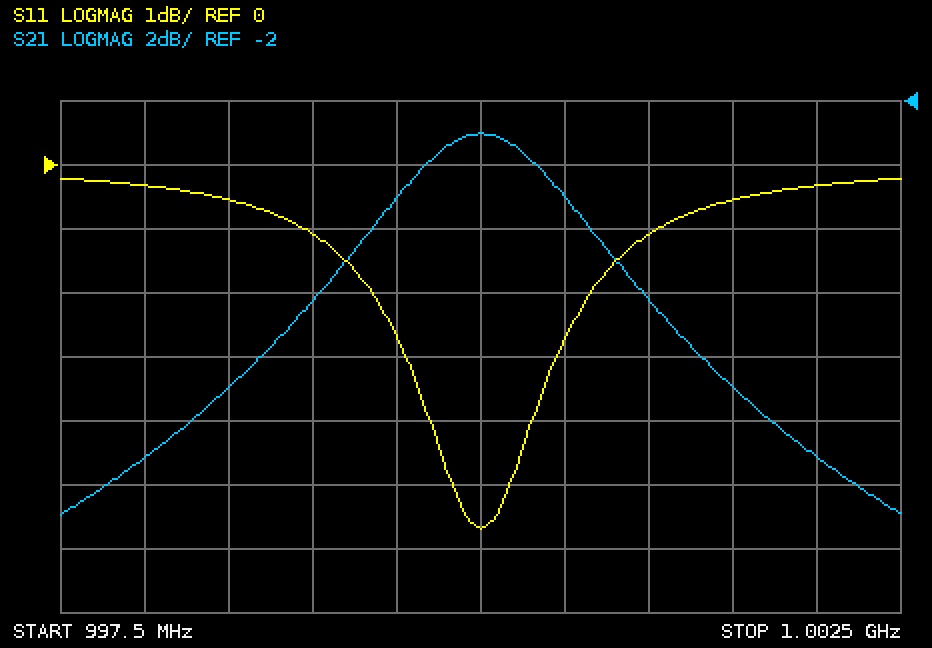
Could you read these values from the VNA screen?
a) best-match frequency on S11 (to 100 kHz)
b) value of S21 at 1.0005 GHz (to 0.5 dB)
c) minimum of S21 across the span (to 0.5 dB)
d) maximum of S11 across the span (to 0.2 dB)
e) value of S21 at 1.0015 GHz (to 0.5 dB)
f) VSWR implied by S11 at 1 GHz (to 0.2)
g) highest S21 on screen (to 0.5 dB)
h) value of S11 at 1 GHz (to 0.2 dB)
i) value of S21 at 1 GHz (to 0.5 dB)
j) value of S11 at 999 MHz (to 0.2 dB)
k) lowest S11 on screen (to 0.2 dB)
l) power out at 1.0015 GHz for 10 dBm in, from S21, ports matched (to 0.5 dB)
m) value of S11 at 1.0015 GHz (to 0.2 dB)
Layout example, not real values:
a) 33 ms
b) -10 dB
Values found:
a) 1.0000 GHz
b) -5.0 dB
c) -15.0 dB
d) -0.2 dB
e) -11.0 dB
f) 3.2
g) -3.0 dB
h) -5.6 dB
i) -3.0 dB
j) -1.0 dB
k) -5.6 dB
l) -1.0 dBm
m) -0.6 dB
